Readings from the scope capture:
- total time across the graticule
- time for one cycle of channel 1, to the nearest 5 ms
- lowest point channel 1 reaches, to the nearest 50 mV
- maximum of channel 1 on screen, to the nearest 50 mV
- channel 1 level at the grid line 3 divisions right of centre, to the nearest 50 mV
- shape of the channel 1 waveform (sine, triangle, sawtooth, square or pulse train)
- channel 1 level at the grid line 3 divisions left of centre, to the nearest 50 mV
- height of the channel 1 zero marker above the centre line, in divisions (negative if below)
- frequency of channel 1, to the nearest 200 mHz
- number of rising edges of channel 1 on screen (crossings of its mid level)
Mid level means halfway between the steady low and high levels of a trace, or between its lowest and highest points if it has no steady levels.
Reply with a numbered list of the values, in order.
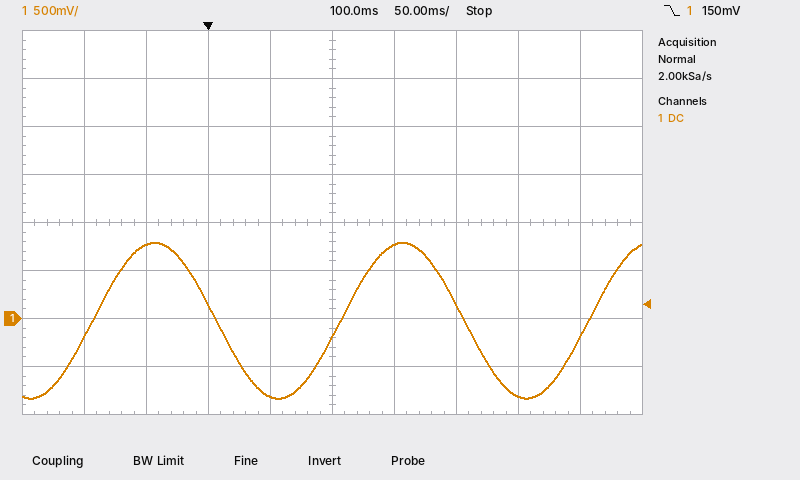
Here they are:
1. 500 ms
2. 200 ms
3. -850 mV
4. 800 mV
5. -800 mV
6. sine
7. 750 mV
8. -2.0 div
9. 5.0 Hz
10. 3
